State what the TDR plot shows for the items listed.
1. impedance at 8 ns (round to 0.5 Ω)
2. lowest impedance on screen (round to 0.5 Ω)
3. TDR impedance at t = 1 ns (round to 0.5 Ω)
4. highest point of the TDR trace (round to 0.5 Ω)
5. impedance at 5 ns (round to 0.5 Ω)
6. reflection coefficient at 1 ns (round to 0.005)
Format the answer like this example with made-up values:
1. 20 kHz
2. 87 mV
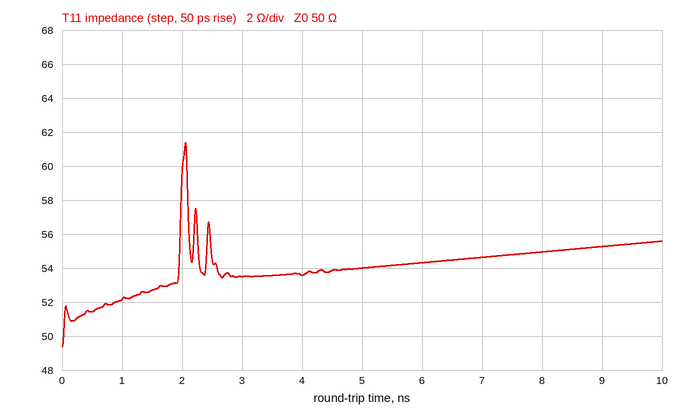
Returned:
1. 55.0 Ω
2. 49.5 Ω
3. 52.0 Ω
4. 61.5 Ω
5. 54.0 Ω
6. +0.020
